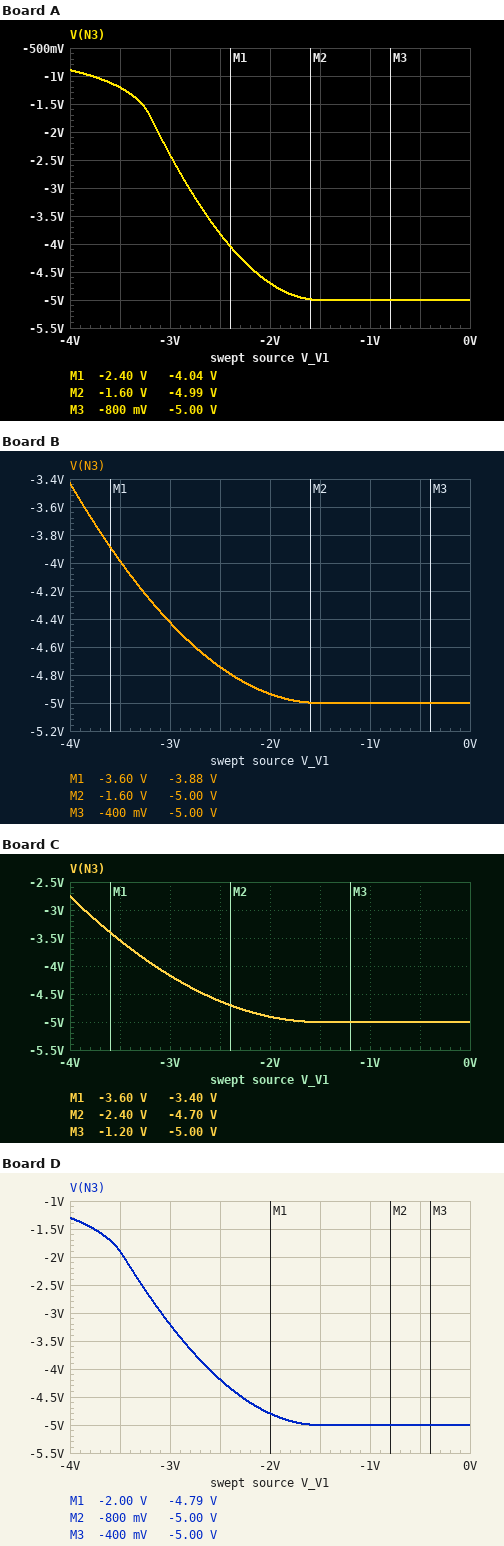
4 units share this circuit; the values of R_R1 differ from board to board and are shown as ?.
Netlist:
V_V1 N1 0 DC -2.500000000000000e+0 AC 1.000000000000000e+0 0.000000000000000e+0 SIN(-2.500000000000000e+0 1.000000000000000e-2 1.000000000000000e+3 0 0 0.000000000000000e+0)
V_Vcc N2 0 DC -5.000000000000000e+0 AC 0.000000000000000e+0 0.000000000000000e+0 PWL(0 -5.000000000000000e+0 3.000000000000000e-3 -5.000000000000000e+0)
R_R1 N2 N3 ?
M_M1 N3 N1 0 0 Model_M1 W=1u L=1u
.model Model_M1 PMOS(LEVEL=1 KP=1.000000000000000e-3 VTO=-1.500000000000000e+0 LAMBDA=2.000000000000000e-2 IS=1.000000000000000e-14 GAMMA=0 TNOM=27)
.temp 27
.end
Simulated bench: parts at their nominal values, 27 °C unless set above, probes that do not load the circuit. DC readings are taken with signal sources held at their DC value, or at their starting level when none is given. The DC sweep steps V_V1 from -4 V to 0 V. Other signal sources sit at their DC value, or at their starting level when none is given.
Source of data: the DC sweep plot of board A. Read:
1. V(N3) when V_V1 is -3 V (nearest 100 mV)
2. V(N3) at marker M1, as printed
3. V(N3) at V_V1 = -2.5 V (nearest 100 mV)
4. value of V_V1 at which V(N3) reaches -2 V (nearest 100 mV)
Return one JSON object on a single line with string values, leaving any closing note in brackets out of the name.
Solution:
{"V(N3) when V_V1 is -3 V": "-2.4 V", "V(N3) at marker M1, as printed": "-4.04 V", "V(N3) at V_V1 = -2.5 V": "-3.8 V", "value of V_V1 at which V(N3) reaches -2 V": "-3.1 V"}
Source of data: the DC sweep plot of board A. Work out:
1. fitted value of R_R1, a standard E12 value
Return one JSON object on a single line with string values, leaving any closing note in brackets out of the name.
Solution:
{"fitted value of R_R1, a standard E12 value": "2.2 kΩ"}
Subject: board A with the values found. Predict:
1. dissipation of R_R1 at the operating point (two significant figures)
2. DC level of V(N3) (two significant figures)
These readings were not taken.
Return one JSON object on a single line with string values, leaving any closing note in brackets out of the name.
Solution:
{"dissipation of R_R1 at the operating point": "640 µW", "DC level of V(N3)": "-3.8 V"}
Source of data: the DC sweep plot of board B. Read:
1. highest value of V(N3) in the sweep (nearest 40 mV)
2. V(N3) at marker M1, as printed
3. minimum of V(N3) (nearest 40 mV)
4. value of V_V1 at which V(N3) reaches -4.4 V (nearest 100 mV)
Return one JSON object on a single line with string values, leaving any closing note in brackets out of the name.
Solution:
{"highest value of V(N3) in the sweep": "-3.44 V", "V(N3) at marker M1, as printed": "-3.88 V", "minimum of V(N3)": "-5.00 V", "value of V_V1 at which V(N3) reaches -4.4 V": "-3.0 V"}
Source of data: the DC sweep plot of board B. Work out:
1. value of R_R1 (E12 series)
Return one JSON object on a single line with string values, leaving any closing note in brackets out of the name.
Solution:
{"value of R_R1": "470 Ω"}
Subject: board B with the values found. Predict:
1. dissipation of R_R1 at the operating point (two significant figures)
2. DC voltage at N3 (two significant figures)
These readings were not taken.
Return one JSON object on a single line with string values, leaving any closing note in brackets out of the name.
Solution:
{"dissipation of R_R1 at the operating point": "140 µW", "DC voltage at N3": "-4.7 V"}
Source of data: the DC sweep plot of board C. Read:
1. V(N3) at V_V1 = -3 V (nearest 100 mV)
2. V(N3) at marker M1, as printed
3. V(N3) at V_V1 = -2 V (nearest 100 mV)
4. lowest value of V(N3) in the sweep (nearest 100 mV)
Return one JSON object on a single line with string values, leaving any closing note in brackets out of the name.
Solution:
{"V(N3) at V_V1 = -3 V": "-4.2 V", "V(N3) at marker M1, as printed": "-3.40 V", "V(N3) at V_V1 = -2 V": "-4.9 V", "lowest value of V(N3) in the sweep": "-5.0 V"}
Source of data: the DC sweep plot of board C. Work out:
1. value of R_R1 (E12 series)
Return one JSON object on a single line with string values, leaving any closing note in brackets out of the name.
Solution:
{"value of R_R1": "680 Ω"}
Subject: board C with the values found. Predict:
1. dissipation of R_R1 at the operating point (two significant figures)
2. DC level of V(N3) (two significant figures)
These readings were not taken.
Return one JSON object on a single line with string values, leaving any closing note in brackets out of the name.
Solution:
{"dissipation of R_R1 at the operating point": "200 µW", "DC level of V(N3)": "-4.6 V"}
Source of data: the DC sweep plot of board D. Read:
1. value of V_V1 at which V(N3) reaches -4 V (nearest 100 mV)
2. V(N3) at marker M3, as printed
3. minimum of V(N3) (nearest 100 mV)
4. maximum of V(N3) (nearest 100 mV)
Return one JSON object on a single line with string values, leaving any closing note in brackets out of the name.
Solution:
{"value of V_V1 at which V(N3) reaches -4 V": "-2.6 V", "V(N3) at marker M3, as printed": "-5.00 V", "minimum of V(N3)": "-5.0 V", "maximum of V(N3)": "-1.3 V"}
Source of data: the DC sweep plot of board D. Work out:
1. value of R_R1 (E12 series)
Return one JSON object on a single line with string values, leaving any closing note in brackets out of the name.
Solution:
{"value of R_R1": "1.5 kΩ"}
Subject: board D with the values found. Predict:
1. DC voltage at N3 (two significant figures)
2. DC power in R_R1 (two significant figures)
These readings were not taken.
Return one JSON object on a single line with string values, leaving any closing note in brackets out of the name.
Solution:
{"DC voltage at N3": "-4.2 V", "DC power in R_R1": "440 µW"}
